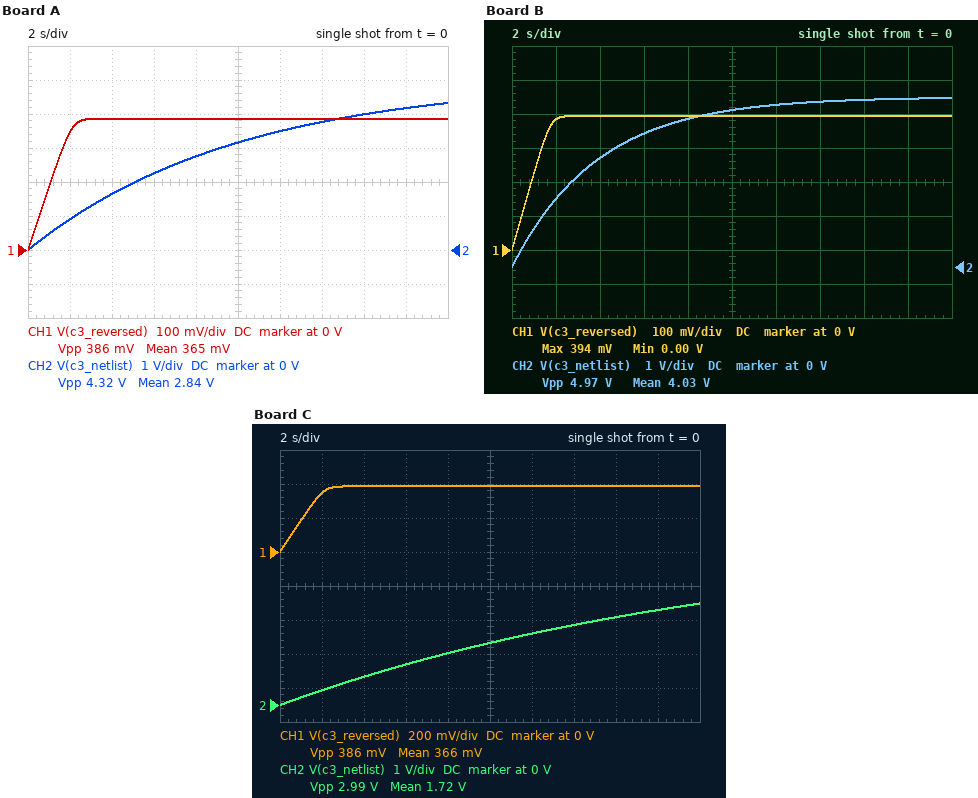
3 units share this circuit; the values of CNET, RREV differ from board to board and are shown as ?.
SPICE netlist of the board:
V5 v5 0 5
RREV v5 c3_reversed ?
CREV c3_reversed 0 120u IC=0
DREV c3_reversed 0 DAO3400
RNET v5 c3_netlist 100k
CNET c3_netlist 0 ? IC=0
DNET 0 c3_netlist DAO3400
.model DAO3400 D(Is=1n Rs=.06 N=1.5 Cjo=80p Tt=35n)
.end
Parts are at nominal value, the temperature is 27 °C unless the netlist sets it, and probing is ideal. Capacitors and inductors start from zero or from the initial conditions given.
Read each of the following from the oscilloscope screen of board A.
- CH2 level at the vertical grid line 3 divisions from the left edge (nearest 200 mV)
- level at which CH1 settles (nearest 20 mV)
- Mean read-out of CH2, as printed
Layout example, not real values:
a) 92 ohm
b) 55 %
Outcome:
a) 2.2 V
b) 380 mV
c) 2.84 V
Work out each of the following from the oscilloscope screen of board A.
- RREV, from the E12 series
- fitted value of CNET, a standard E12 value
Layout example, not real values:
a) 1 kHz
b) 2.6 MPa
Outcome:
a) 220 kΩ
b) 100 µF
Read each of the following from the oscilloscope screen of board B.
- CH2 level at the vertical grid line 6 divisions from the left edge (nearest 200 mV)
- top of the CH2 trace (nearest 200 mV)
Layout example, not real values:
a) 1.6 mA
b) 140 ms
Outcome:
a) 4.8 V
b) 5.0 V
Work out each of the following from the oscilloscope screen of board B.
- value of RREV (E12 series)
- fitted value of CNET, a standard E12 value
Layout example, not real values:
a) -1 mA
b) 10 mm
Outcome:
a) 180 kΩ
b) 39 µF
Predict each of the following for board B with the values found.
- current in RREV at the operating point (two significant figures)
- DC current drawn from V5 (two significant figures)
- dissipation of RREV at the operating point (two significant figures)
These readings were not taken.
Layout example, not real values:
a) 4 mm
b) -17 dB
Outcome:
a) 26 µA
b) 26 µA
c) 120 µW
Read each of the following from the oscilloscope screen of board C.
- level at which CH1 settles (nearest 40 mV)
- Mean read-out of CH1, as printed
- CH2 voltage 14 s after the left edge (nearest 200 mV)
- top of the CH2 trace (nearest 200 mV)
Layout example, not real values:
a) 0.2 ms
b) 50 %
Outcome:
a) 400 mV
b) 366 mV
c) 2.4 V
d) 3.0 V
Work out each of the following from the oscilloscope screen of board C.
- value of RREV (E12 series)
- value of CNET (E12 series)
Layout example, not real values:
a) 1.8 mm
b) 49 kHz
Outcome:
a) 220 kΩ
b) 220 µF
